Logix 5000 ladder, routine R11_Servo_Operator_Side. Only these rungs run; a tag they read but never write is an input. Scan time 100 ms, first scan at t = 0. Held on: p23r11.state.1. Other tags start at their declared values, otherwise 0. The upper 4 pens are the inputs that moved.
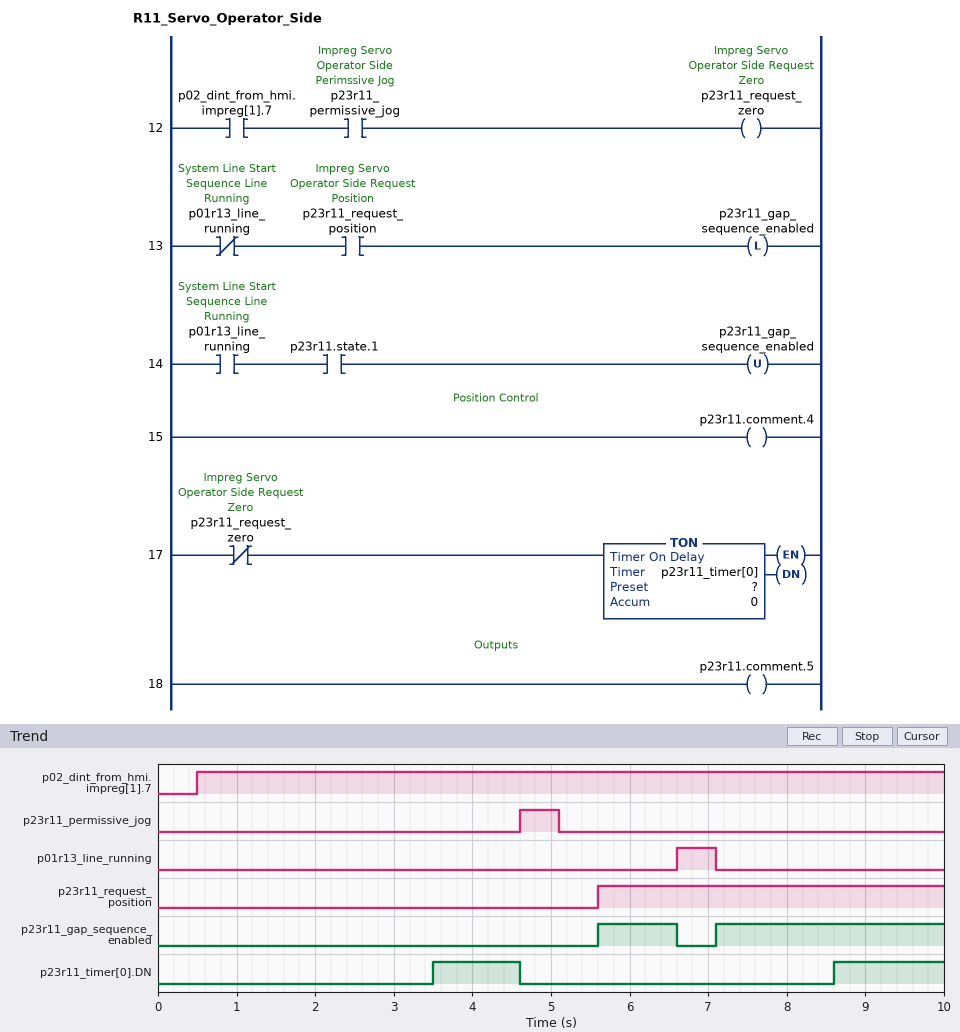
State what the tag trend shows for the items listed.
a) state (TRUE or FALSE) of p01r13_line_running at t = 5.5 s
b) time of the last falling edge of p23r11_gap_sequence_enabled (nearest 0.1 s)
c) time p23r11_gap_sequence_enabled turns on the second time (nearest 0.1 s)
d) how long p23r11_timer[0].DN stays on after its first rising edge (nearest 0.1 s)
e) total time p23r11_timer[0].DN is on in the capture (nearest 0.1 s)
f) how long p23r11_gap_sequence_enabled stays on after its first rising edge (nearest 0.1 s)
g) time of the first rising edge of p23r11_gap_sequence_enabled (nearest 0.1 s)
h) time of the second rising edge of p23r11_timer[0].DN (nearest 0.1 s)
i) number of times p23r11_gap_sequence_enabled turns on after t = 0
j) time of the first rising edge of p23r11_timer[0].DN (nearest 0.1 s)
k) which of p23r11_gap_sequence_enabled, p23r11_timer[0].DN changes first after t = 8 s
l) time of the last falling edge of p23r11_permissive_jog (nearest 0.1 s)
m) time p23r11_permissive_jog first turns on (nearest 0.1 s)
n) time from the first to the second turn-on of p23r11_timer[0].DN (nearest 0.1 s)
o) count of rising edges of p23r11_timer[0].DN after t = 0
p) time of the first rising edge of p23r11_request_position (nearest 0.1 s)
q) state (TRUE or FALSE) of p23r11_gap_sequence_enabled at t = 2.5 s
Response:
FALSE
6.6 s
7.1 s
1.1 s
2.5 s
1.0 s
5.6 s
8.6 s
2
3.5 s
p23r11_timer[0].DN
5.1 s
4.6 s
5.1 s
2
5.6 s
FALSE
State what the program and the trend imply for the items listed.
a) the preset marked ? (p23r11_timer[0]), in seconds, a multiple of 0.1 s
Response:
3.5 s
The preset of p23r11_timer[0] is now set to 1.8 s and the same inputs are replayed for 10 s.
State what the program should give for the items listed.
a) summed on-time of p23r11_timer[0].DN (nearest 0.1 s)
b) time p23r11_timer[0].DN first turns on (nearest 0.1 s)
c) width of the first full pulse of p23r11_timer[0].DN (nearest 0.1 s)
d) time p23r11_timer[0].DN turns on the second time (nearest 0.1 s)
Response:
5.9 s
1.8 s
2.8 s
6.9 s
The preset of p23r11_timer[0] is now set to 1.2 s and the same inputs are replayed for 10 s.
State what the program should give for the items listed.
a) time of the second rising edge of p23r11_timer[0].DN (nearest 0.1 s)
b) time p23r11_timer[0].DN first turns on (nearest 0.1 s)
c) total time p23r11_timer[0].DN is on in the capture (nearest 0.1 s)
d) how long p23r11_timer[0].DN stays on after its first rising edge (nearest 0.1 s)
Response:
6.3 s
1.2 s
7.1 s
3.4 s
